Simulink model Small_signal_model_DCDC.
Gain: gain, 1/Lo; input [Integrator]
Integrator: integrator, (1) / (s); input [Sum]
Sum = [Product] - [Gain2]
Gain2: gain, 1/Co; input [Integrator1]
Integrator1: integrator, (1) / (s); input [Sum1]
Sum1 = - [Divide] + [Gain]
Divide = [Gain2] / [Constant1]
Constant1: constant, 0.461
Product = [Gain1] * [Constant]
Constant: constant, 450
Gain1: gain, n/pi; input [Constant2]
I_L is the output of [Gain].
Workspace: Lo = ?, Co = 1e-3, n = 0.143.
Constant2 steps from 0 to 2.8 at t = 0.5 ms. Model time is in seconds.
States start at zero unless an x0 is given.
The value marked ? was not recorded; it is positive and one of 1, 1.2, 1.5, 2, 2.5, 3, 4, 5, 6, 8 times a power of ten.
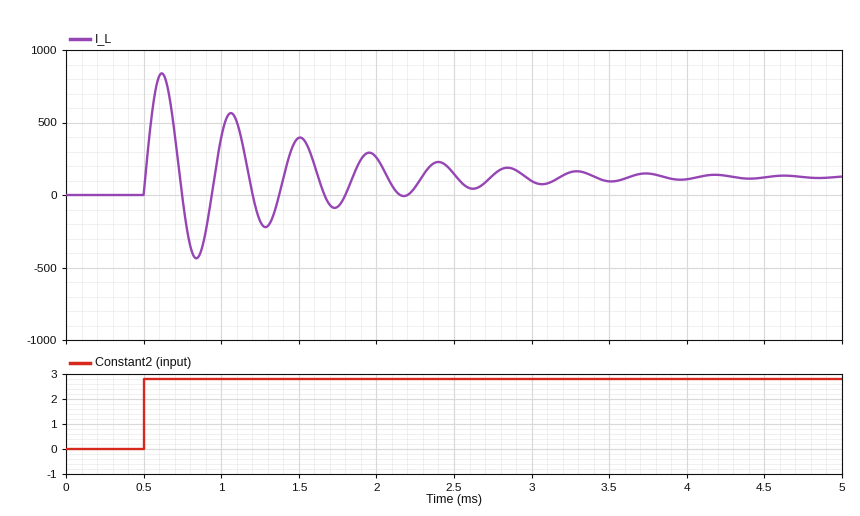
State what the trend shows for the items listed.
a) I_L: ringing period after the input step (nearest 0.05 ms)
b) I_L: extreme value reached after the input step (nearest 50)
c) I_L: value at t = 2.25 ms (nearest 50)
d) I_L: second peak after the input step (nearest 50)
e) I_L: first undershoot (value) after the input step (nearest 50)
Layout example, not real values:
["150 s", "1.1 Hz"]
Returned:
["0.45 ms", "850", "50", "550", "-450"]
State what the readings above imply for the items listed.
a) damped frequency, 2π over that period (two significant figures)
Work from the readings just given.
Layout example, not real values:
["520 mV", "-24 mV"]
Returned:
["14 rad/ms"]
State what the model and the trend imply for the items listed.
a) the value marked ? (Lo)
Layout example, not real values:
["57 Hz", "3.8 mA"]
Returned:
["5e-06"]
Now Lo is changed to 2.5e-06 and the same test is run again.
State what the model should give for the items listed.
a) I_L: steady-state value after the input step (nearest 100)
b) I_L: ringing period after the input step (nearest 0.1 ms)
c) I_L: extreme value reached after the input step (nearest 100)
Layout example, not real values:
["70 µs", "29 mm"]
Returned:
["100", "0.3 ms", "1200"]
